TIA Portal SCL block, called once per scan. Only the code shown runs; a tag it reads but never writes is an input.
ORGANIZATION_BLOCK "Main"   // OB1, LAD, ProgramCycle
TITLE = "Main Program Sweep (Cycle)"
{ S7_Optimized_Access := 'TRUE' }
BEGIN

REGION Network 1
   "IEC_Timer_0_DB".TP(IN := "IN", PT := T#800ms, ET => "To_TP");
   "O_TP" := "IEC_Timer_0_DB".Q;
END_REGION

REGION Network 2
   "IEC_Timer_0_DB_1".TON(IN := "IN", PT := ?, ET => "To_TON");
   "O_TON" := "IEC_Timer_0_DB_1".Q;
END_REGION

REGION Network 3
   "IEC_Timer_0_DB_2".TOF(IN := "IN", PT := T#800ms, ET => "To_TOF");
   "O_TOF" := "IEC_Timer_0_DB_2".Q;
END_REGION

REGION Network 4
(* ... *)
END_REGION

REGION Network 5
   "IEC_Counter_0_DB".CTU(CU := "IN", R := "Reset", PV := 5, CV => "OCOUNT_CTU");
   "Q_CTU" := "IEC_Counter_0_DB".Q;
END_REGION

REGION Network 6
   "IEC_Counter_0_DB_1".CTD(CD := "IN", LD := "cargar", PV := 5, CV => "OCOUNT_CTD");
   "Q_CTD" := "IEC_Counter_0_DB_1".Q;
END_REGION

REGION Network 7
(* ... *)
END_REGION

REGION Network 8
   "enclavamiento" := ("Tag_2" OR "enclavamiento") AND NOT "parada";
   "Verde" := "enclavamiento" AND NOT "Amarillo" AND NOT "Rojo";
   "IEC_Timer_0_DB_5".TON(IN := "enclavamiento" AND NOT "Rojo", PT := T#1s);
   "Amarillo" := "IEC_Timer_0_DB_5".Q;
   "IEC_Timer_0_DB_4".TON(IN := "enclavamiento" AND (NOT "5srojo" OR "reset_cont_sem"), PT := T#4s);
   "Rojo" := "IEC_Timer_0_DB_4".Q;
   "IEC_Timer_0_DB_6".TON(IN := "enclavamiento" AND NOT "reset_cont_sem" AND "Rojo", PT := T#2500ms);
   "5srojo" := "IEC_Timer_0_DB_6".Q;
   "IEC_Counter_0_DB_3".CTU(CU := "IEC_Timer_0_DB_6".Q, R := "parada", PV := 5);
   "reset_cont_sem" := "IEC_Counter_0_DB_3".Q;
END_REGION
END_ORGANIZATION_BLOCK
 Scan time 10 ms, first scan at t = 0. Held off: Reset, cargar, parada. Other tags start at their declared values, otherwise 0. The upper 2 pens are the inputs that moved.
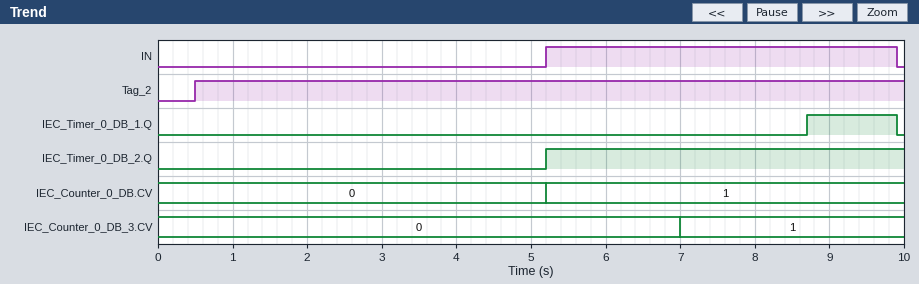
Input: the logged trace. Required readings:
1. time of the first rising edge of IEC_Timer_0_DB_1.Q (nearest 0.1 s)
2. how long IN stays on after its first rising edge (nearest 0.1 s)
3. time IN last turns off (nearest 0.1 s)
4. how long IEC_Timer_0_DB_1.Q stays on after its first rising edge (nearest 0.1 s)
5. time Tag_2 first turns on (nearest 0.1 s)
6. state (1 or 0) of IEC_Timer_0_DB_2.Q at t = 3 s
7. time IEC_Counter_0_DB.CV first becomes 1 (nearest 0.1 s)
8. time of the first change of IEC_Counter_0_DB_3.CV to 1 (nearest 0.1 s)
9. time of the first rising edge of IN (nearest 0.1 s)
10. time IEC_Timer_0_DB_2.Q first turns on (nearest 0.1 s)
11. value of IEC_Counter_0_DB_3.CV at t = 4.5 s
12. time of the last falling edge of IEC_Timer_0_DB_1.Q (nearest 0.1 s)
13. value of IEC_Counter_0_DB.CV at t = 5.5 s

8.7 s
4.7 s
9.9 s
1.2 s
0.5 s
0
5.2 s
7.0 s
5.2 s
5.2 s
0
9.9 s
1
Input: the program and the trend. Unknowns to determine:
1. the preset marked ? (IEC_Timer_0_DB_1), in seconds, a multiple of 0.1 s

3.5 s
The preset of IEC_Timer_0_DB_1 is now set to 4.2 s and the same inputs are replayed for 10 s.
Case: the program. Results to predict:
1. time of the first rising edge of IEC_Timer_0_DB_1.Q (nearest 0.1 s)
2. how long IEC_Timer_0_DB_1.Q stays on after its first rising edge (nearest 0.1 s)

9.4 s
0.5 s
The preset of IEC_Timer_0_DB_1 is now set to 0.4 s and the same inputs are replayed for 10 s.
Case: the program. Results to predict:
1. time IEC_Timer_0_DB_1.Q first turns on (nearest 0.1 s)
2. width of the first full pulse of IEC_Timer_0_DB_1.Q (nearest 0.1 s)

5.6 s
4.3 s
